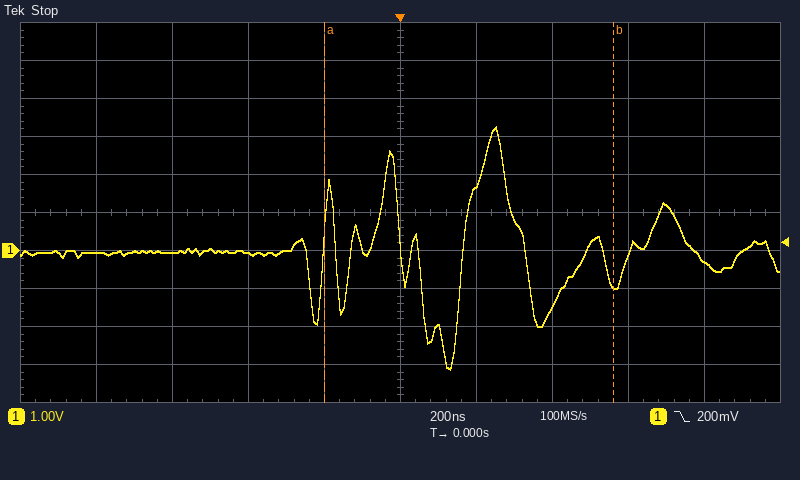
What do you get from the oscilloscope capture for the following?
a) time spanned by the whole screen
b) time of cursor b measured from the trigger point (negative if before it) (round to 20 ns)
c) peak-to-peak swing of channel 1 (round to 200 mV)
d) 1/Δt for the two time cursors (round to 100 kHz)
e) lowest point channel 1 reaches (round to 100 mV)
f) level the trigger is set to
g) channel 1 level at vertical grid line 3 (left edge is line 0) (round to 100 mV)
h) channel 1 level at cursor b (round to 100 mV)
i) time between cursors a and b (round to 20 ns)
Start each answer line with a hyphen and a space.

- 2 µs
- +560 ns
- 6.4 V
- 1.3 MHz
- -3.1 V
- 200 mV
- -100 mV
- -900 mV
- 760 ns
